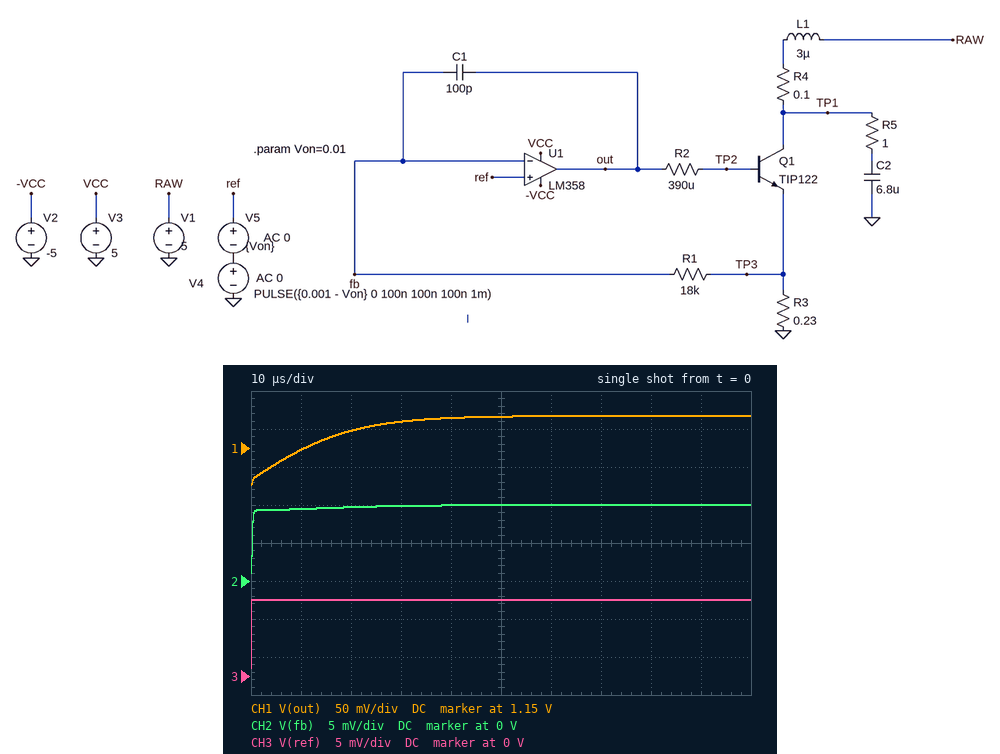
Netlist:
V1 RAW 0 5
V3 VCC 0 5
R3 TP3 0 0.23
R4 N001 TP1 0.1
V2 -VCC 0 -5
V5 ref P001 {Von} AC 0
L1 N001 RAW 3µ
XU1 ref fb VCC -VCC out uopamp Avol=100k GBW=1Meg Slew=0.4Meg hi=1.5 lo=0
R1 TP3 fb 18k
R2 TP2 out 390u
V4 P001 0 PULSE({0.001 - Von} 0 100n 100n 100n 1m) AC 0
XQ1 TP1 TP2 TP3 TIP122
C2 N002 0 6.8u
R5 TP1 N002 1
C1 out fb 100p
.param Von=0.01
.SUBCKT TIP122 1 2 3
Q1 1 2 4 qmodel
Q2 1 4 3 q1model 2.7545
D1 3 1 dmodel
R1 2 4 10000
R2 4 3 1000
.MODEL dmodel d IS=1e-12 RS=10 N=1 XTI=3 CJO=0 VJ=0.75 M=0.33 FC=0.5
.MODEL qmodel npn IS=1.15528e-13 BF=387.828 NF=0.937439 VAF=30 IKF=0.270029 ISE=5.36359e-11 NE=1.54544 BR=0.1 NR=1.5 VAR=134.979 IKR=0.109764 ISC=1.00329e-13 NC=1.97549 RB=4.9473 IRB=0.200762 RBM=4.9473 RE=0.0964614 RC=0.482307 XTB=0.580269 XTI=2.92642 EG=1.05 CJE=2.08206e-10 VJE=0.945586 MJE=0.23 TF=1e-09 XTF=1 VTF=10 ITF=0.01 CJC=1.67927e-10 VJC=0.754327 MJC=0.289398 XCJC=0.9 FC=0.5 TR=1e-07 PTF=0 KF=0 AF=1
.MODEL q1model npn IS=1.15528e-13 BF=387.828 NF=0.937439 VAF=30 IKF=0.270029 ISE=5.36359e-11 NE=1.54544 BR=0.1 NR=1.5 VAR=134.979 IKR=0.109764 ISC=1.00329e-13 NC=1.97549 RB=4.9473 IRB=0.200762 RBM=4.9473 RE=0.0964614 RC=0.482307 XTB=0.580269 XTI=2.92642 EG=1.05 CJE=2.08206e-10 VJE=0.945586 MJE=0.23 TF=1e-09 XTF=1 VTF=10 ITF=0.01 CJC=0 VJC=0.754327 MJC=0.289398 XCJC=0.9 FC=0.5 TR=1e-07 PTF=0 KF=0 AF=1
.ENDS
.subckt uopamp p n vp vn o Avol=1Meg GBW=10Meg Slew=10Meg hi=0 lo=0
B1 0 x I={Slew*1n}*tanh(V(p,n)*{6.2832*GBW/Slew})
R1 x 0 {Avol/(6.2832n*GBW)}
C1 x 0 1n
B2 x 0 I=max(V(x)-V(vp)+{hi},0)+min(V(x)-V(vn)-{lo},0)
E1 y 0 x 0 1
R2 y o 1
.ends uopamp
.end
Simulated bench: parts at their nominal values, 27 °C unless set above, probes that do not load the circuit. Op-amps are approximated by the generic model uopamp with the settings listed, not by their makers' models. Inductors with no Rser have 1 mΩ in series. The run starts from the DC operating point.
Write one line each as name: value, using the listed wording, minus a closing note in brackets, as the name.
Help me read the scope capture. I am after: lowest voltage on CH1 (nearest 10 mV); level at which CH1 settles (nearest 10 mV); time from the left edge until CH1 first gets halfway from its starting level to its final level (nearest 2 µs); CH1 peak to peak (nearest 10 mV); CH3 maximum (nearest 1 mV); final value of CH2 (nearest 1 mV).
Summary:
lowest voltage on CH1: 1.10 V
level at which CH1 settles: 1.19 V
time from the left edge until CH1 first gets halfway from its starting level to its final level: 10 µs
CH1 peak to peak: 90 mV
CH3 maximum: 10 mV
final value of CH2: 10 mV
